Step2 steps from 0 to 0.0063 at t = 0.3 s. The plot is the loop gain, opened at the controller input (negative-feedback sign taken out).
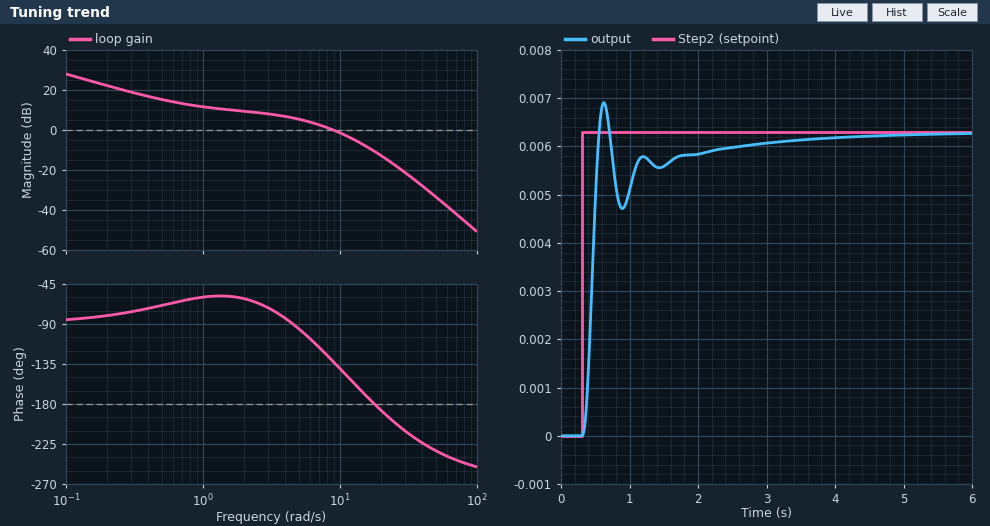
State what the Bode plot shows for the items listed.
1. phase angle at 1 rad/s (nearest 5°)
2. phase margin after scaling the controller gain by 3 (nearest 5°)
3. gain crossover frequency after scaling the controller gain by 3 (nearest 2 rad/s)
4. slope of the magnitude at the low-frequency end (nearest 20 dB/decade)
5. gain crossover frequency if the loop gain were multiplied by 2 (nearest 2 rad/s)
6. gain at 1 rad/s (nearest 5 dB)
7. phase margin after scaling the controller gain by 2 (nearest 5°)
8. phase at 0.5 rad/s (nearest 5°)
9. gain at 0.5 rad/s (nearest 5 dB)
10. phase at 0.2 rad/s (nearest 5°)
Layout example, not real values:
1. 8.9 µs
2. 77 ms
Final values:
1. -60°
2. 5°
3. 16 rad/s
4. -20 dB/decade
5. 14 rad/s
6. 10 dB
7. 20°
8. -70°
9. 15 dB
10. -80°
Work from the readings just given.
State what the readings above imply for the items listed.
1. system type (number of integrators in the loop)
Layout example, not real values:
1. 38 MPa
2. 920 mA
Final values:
1. 1
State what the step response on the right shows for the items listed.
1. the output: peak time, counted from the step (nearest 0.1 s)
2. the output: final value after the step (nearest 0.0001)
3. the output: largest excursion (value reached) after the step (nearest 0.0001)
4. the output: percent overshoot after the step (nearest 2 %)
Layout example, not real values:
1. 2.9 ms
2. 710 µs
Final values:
1. 0.3 s
2. 0.0063
3. 0.0069
4. 10 %
